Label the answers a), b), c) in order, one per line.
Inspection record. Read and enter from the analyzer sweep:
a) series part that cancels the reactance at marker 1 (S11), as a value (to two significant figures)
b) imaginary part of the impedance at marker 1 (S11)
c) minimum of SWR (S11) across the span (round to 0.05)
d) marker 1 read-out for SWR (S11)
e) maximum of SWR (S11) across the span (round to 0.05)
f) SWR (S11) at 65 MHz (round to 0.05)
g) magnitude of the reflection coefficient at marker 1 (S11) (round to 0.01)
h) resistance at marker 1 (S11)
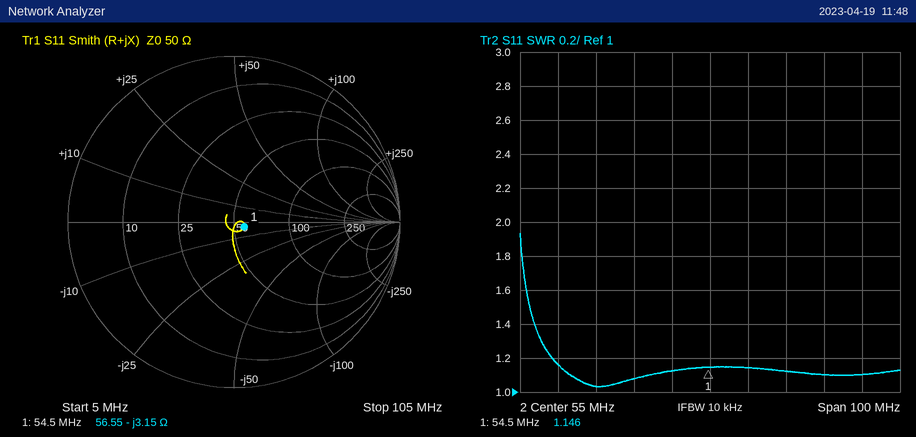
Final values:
a) 9.2 nH
b) -3.15 Ω
c) 1.05
d) 1.146
e) 1.95
f) 1.15
g) 0.07
h) 56.55 Ω
